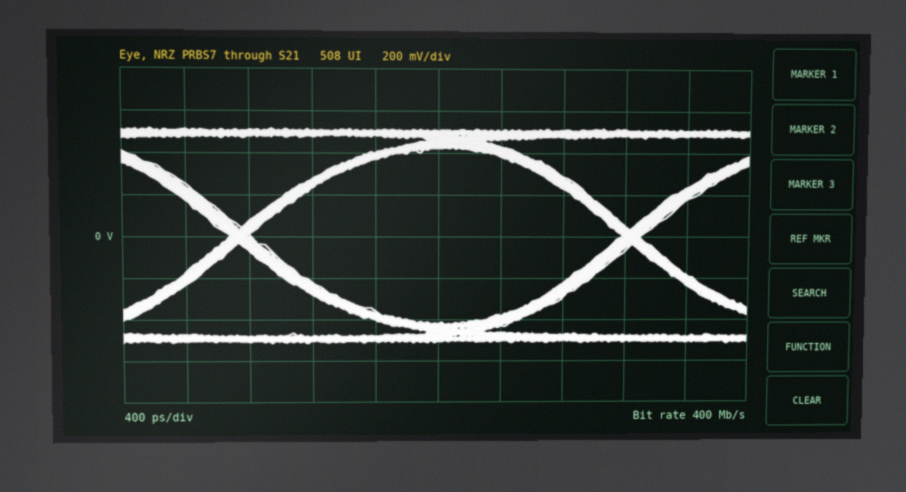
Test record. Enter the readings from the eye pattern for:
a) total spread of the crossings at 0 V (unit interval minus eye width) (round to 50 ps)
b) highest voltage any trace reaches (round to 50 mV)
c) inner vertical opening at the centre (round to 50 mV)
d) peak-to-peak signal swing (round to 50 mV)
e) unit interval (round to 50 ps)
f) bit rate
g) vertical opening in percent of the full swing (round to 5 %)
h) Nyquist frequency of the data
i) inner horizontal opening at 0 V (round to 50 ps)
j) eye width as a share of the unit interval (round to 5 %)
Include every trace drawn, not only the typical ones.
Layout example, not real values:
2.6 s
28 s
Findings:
150 ps
500 mV
850 mV
1.05 V
2.50 ns
400 Mb/s
80 %
200 MHz
2.35 ns
95 %
